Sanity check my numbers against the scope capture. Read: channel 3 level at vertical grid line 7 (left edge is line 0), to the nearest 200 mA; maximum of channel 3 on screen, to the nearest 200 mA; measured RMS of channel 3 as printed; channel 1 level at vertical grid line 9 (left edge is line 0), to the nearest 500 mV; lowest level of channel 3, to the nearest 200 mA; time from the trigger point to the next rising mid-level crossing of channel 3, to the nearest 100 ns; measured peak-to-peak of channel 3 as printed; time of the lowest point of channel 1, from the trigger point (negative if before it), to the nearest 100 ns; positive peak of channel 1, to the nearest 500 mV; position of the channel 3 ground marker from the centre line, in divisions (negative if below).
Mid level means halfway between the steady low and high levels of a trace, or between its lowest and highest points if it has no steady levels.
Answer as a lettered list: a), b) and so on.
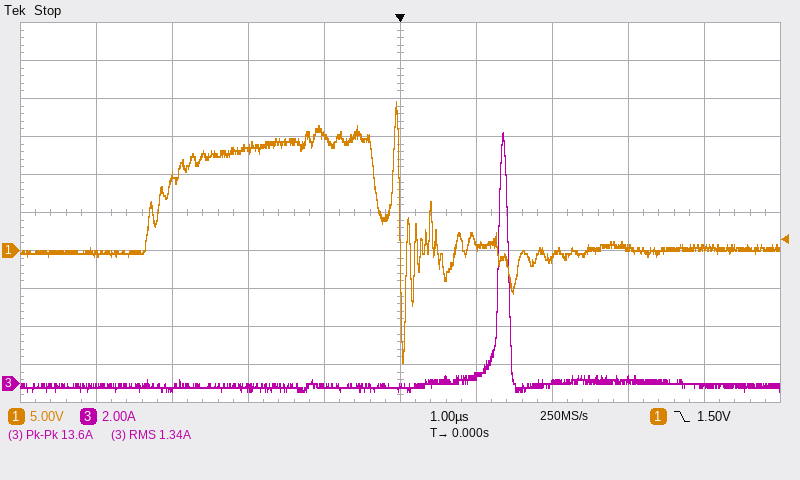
a) 0.0 A
b) 13.2 A
c) 1.34 A
d) 500 mV
e) -400 mA
f) 1.3 µs
g) 13.6 A
h) 0.0 µs
i) 19.5 V
j) -4.5 div
